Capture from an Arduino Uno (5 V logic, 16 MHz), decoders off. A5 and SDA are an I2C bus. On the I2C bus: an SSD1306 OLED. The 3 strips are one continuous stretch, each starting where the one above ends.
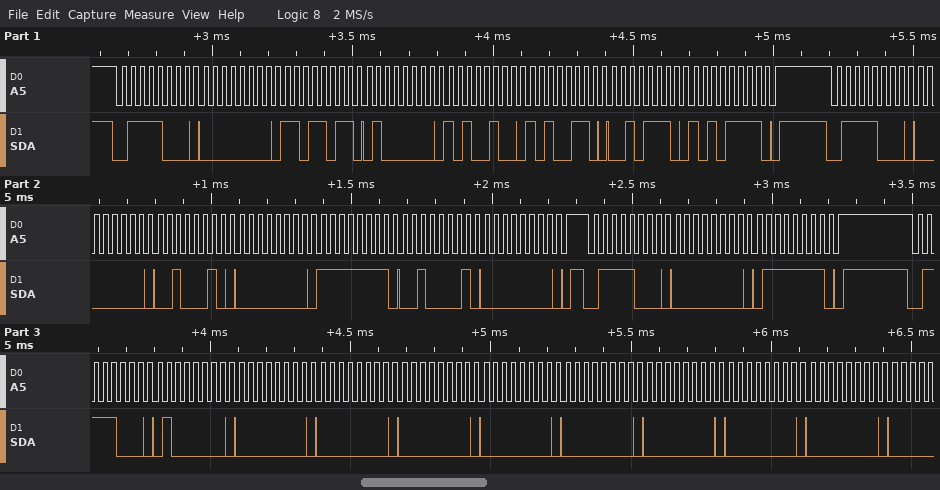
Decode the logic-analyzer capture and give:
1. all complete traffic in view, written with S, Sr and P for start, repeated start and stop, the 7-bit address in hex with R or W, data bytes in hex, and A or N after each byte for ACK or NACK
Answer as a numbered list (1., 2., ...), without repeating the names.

1. S 3CW A 00 A DB A 40 A A4 A A6 A 2E A AF A P S 3CW A 00 A 22 A 00 A FF A 21 A 00 A P S 3CW A 00 A 7F A P S 3CW A 40 A 00 A 00 A 00 A 00 A 00 A 00 A 00 A 00 A
